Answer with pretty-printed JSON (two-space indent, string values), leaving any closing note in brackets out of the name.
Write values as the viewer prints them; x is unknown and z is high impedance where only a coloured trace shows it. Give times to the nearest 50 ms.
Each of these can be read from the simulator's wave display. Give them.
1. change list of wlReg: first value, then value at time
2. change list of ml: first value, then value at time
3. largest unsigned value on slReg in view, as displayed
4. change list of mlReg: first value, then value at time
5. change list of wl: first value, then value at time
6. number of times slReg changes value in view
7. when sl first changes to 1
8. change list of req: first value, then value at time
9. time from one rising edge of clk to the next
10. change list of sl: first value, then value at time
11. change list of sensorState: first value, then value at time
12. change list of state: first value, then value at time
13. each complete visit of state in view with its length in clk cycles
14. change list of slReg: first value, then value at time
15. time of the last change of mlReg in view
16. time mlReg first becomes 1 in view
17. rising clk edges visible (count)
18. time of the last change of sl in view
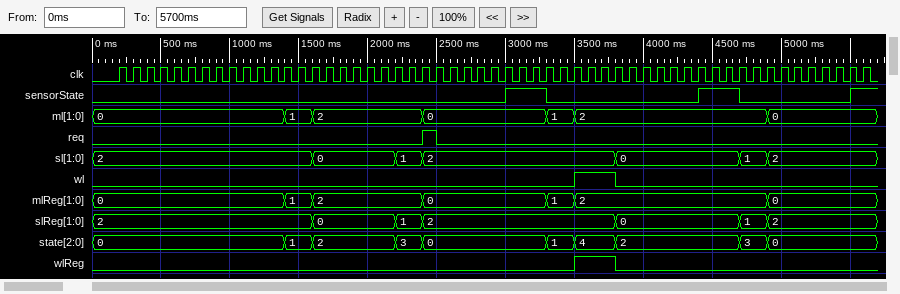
{
  "change list of wlReg: first value, then value at time": "0, 1 at 3500 ms, 0 at 3800 ms",
  "change list of ml: first value, then value at time": "0, 1 at 1400 ms, 2 at 1600 ms, 0 at 2400 ms, 1 at 3300 ms, 2 at 3500 ms, 0 at 4900 ms",
  "largest unsigned value on slReg in view, as displayed": "2",
  "change list of mlReg: first value, then value at time": "0, 1 at 1400 ms, 2 at 1600 ms, 0 at 2400 ms, 1 at 3300 ms, 2 at 3500 ms, 0 at 4900 ms",
  "change list of wl: first value, then value at time": "0, 1 at 3500 ms, 0 at 3800 ms",
  "number of times slReg changes value in view": "6",
  "when sl first changes to 1": "2200 ms",
  "change list of req: first value, then value at time": "0, 1 at 2400 ms, 0 at 2500 ms",
  "time from one rising edge of clk to the next": "100 ms",
  "change list of sl: first value, then value at time": "2, 0 at 1600 ms, 1 at 2200 ms, 2 at 2400 ms, 0 at 3800 ms, 1 at 4700 ms, 2 at 4900 ms",
  "change list of sensorState: first value, then value at time": "0, 1 at 3000 ms, 0 at 3300 ms, 1 at 4400 ms, 0 at 4700 ms, 1 at 5500 ms",
  "change list of state: first value, then value at time": "0, 1 at 1400 ms, 2 at 1600 ms, 3 at 2200 ms, 0 at 2400 ms, 1 at 3300 ms, 4 at 3500 ms, 2 at 3800 ms, 3 at 4700 ms, 0 at 4900 ms",
  "each complete visit of state in view with its length in clk cycles": "1: 2, 2: 6, 3: 2, 0: 9, 1: 2, 4: 3, 2: 9, 3: 2",
  "change list of slReg: first value, then value at time": "2, 0 at 1600 ms, 1 at 2200 ms, 2 at 2400 ms, 0 at 3800 ms, 1 at 4700 ms, 2 at 4900 ms",
  "time of the last change of mlReg in view": "4900 ms",
  "time mlReg first becomes 1 in view": "1400 ms",
  "rising clk edges visible": "55",
  "time of the last change of sl in view": "4900 ms"
}
